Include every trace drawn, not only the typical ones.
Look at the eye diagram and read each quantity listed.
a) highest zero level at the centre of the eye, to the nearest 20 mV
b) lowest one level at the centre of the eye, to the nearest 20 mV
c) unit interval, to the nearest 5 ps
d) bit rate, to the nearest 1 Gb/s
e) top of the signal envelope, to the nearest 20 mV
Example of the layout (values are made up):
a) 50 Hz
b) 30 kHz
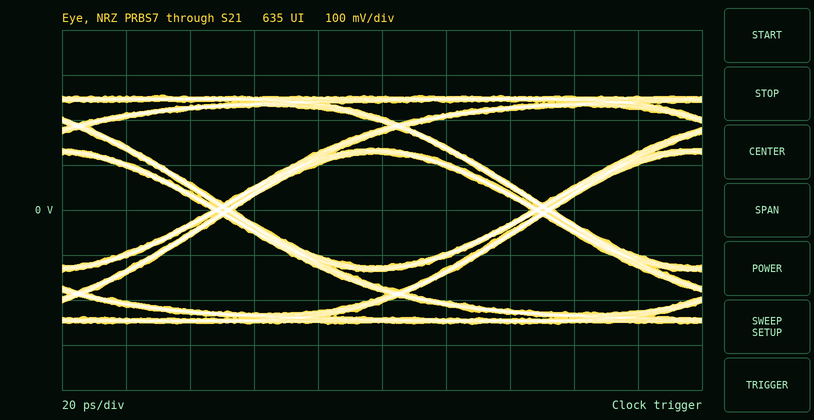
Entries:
a) -120 mV
b) 120 mV
c) 100 ps
d) 10 Gb/s
e) 260 mV
